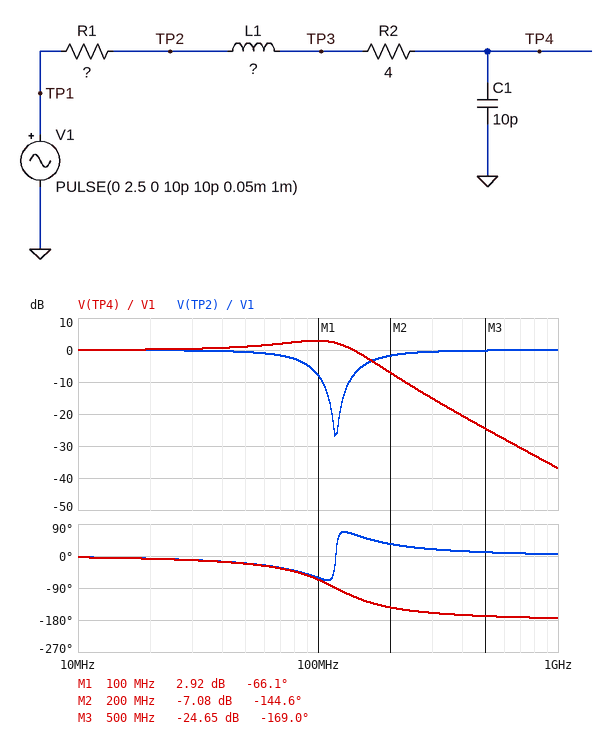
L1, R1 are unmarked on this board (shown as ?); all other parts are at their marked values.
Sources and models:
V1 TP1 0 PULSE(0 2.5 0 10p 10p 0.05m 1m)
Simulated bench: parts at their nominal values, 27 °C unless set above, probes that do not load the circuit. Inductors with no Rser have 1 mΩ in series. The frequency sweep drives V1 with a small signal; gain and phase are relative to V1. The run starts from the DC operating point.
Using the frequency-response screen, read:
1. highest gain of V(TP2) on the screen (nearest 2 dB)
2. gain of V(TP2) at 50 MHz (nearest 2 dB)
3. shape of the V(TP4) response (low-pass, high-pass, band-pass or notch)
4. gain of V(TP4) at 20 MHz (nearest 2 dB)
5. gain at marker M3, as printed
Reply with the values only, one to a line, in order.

0 dB
0 dB
low-pass
0 dB
-24.65 dB
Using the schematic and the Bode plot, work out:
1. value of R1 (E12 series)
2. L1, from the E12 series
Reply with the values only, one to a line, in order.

100 Ω
180 nH
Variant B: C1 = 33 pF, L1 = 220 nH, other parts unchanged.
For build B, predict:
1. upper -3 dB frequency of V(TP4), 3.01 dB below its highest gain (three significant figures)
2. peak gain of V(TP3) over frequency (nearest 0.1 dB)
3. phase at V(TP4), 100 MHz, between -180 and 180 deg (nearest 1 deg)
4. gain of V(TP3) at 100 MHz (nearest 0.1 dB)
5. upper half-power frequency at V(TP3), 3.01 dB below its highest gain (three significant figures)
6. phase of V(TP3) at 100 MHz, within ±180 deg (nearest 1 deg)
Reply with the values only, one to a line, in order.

63.9 MHz
0.2 dB
-131 deg
-9.1 dB
64.0 MHz
-126 deg
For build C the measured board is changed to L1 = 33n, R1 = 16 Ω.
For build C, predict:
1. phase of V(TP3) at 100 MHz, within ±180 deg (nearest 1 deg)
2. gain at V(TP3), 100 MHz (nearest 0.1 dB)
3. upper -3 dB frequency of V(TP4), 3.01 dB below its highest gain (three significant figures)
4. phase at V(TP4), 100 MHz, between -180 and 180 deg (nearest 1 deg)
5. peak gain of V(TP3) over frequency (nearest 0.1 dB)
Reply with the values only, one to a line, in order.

-7 deg
1.1 dB
314 MHz
-8 deg
9.3 dB
